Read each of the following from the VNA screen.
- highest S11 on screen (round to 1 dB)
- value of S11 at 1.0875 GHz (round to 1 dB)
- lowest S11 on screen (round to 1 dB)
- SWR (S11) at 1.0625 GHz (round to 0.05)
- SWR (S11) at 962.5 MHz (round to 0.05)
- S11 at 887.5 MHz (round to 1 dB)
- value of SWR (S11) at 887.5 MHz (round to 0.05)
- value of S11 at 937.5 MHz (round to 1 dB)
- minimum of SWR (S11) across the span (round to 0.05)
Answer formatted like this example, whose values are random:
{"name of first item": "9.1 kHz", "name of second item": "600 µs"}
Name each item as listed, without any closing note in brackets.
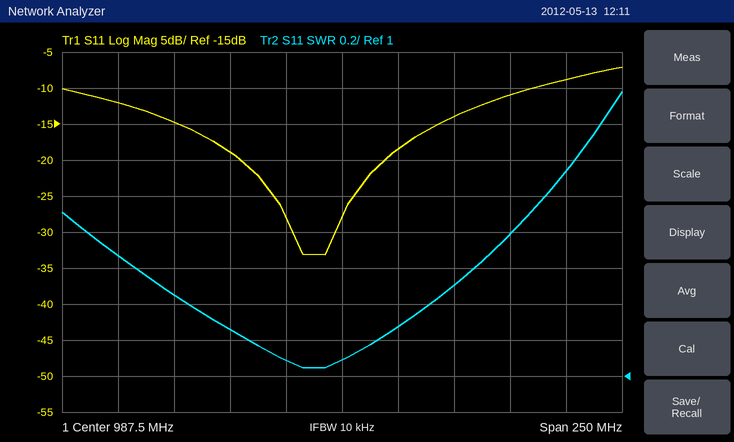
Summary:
{"highest S11 on screen": "-7 dB", "value of S11 at 1.0875 GHz": "-9 dB", "lowest S11 on screen": "-33 dB", "SWR (S11) at 1.0625 GHz": "1.80", "SWR (S11) at 962.5 MHz": "1.10", "S11 at 887.5 MHz": "-12 dB", "value of SWR (S11) at 887.5 MHz": "1.65", "value of S11 at 937.5 MHz": "-19 dB", "minimum of SWR (S11) across the span": "1.05"}
